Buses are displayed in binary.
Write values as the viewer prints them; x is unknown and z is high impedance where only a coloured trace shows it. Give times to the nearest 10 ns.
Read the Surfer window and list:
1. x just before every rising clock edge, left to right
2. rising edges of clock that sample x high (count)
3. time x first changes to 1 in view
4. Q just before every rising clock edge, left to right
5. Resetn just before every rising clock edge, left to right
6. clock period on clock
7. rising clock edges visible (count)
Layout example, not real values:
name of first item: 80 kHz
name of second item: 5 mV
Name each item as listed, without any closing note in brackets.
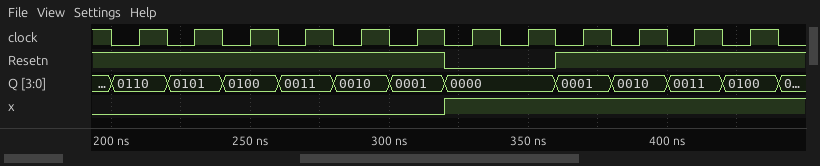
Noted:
x just before every rising clock edge, left to right: 0 0 0 0 0 0 1 1 1 1 1 1
rising edges of clock that sample x high: 6
time x first changes to 1 in view: 320 ns
Q just before every rising clock edge, left to right: 0110, 0101, 0100, 0011, 0010, 0001, 0000, 0000, 0001, 0010, 0011, 0100
Resetn just before every rising clock edge, left to right: 1 1 1 1 1 1 0 0 1 1 1 1
clock period on clock: 20 ns
rising clock edges visible: 12
